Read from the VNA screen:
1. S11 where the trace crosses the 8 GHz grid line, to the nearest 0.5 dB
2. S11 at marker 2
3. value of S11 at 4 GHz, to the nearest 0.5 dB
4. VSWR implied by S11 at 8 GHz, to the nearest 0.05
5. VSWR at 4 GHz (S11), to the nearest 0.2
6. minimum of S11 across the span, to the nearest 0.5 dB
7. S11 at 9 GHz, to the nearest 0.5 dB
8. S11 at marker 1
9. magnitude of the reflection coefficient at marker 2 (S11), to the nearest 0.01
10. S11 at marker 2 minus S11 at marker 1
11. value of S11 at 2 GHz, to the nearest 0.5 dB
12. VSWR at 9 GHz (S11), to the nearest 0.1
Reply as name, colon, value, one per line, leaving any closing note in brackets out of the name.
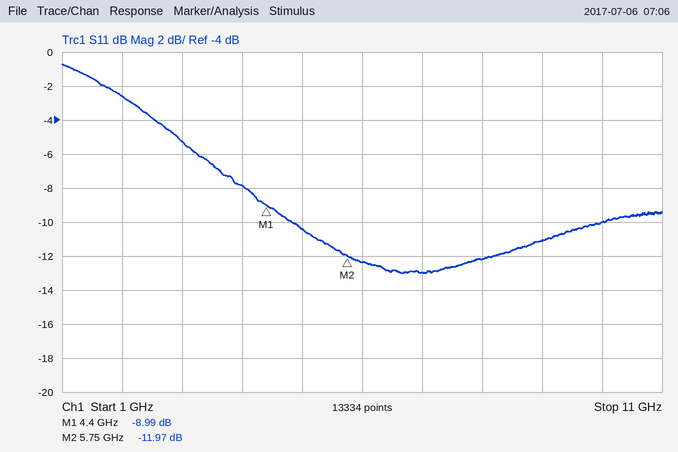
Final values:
S11 where the trace crosses the 8 GHz grid line, to the nearest 0.5 dB: -12.0 dB
S11 at marker 2: -11.97 dB
value of S11 at 4 GHz, to the nearest 0.5 dB: -8.0 dB
VSWR implied by S11 at 8 GHz, to the nearest 0.05: 1.65
VSWR at 4 GHz (S11), to the nearest 0.2: 2.4
minimum of S11 across the span, to the nearest 0.5 dB: -13.0 dB
S11 at 9 GHz, to the nearest 0.5 dB: -11.0 dB
S11 at marker 1: -8.99 dB
magnitude of the reflection coefficient at marker 2 (S11), to the nearest 0.01: 0.25
S11 at marker 2 minus S11 at marker 1: -2.98 dB
value of S11 at 2 GHz, to the nearest 0.5 dB: -2.5 dB
VSWR at 9 GHz (S11), to the nearest 0.1: 1.8
